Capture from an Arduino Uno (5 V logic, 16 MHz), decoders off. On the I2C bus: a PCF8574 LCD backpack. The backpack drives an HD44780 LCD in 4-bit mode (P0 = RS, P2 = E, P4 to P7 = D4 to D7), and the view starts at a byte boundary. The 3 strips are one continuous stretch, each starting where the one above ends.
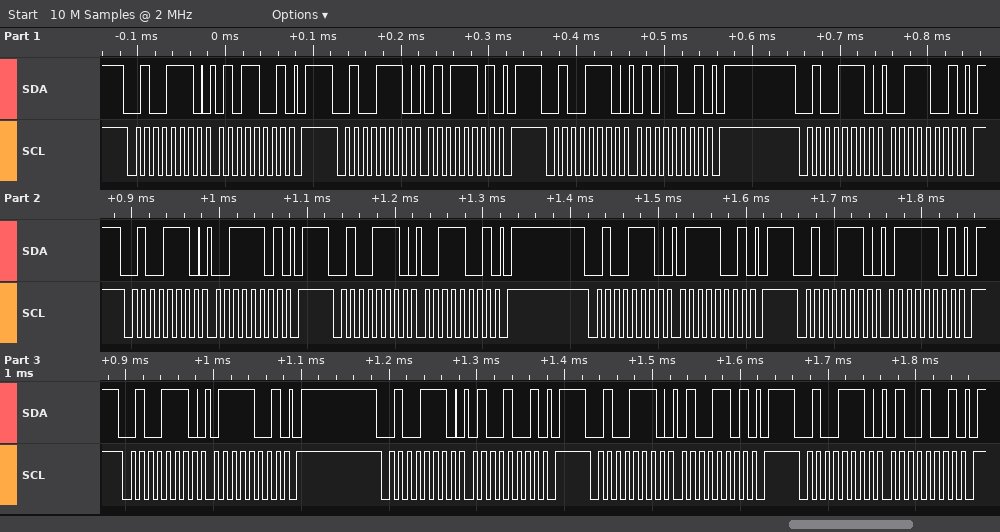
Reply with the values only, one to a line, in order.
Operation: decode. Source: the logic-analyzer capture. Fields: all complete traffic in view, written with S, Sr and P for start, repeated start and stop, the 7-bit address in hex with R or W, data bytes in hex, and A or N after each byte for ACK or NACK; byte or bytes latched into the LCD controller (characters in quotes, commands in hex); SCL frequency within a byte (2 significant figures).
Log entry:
S 27W A 59 A P S 27W A 5D A P S 27W A 59 A P S 27W A 39 A P S 27W A 3D A P S 27W A 39 A P S 27W A 79 A P S 27W A 7D A P S 27W A 79 A P S 27W A 49 A P S 27W A 4D A P S 27W A 49 A P
'S' 't'
100 kHz
